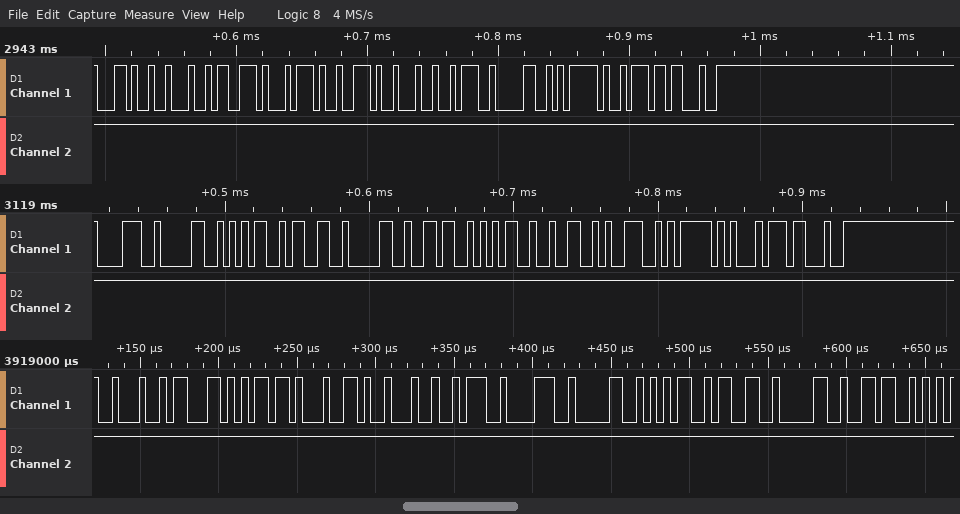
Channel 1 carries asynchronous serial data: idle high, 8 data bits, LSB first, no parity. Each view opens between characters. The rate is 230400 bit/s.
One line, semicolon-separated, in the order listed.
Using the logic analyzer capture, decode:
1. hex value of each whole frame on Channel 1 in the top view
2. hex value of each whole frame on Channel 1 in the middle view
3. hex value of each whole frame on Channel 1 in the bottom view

2C, 22, 73, 74, 72, 22, 3A, 30, 7D, BA, 23; 38, 30, 35, 33, 30, 36, 35, 32, 39, 7D, D1, 23; 22, 63, 6D, 64, 22, 3A, 38, 30, 35, 33, 30, 36
